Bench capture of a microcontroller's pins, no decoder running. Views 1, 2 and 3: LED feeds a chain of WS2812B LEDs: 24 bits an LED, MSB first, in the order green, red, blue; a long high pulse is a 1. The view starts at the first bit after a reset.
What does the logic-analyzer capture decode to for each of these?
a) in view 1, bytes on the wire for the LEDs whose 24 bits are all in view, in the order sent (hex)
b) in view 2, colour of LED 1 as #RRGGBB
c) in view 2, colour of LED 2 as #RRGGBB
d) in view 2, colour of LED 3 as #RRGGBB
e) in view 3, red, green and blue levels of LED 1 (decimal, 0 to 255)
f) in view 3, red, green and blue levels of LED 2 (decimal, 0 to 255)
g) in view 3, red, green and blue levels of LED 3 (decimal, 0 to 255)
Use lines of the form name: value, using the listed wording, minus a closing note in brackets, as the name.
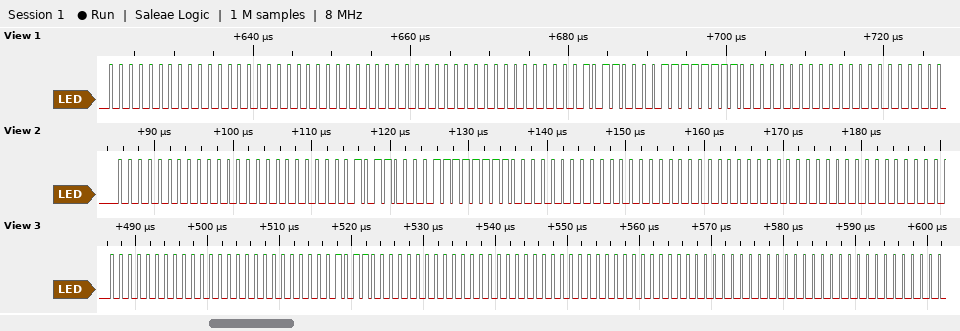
in view 1, bytes on the wire for the LEDs whose 24 bits are all in view, in the order sent: 00 00 00 00 00 00 B0 FF 00
in view 2, colour of LED 1 as #RRGGBB: #000000
in view 2, colour of LED 2 as #RRGGBB: #FFB000
in view 2, colour of LED 3 as #RRGGBB: #000000
in view 3, red, green and blue levels of LED 1: 0, 0, 0
in view 3, red, green and blue levels of LED 2: 0, 88, 0
in view 3, red, green and blue levels of LED 3: 0, 0, 0
